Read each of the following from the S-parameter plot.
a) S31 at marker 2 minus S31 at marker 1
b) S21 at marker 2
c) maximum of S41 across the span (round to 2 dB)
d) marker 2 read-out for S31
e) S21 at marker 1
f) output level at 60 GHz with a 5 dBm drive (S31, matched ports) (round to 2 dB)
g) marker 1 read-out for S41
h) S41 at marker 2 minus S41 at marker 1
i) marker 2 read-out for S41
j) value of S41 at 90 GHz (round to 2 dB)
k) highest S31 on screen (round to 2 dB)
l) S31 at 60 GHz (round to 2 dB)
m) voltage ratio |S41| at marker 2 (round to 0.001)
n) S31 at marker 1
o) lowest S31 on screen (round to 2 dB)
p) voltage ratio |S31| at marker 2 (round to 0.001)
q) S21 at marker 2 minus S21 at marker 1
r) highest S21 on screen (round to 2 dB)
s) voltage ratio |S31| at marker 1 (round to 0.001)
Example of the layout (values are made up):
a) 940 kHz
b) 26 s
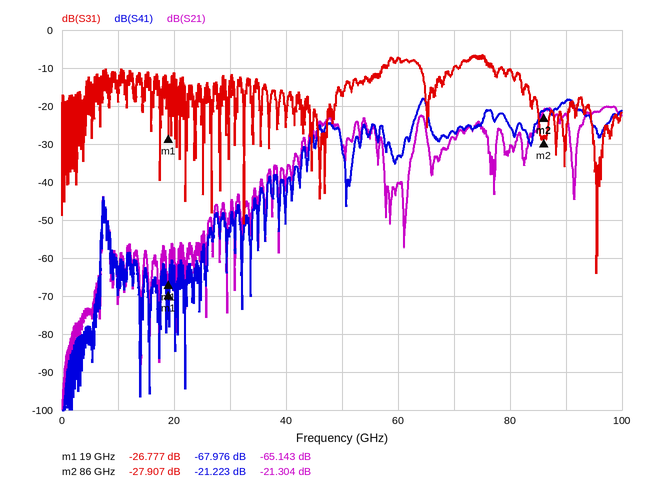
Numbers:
a) -1.130 dB
b) -21.304 dB
c) -18 dB
d) -27.907 dB
e) -65.143 dB
f) -2 dBm
g) -67.976 dB
h) 46.753 dB
i) -21.223 dB
j) -18 dB
k) -6 dB
l) -8 dB
m) 0.087
n) -26.777 dB
o) -64 dB
p) 0.040
q) 43.839 dB
r) -20 dB
s) 0.046
